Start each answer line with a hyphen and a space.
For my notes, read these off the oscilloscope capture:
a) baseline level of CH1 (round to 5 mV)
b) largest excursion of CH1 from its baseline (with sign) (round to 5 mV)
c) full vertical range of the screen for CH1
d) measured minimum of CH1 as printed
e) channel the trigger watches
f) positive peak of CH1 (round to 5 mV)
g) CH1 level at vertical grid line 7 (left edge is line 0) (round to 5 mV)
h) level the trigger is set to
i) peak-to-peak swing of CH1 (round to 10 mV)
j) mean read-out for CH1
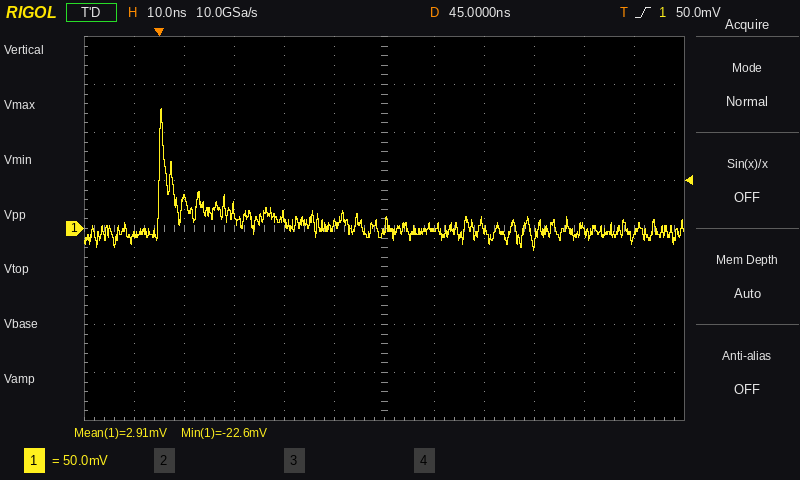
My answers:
- 0 mV
- +125 mV
- 400 mV
- -22.6 mV
- CH1
- 125 mV
- 0 mV
- 50.0 mV
- 150 mV
- 2.91 mV
